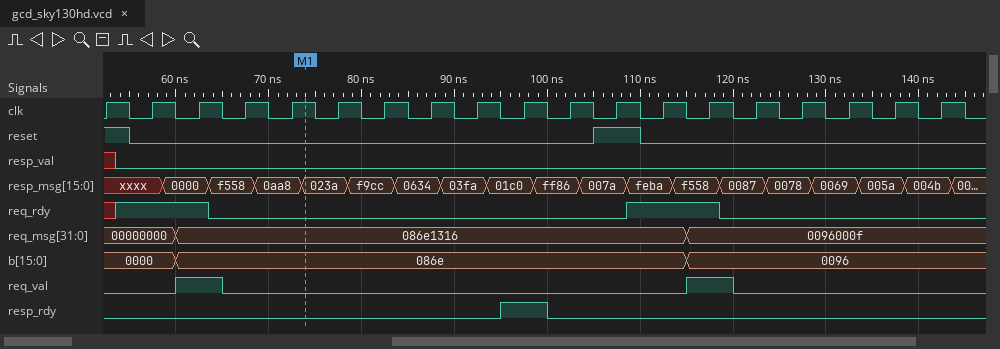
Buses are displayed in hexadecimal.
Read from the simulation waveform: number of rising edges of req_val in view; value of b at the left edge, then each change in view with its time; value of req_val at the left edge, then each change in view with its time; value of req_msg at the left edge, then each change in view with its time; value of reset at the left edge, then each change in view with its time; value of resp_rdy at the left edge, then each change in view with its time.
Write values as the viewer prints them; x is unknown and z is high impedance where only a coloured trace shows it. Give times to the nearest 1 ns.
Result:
2
0000, 086e at 60 ns, 0096 at 115 ns
0, 1 at 60 ns, 0 at 65 ns, 1 at 115 ns, 0 at 120 ns
00000000, 086e1316 at 60 ns, 0096000f at 115 ns
1, 0 at 55 ns, 1 at 105 ns, 0 at 110 ns
0, 1 at 95 ns, 0 at 100 ns
